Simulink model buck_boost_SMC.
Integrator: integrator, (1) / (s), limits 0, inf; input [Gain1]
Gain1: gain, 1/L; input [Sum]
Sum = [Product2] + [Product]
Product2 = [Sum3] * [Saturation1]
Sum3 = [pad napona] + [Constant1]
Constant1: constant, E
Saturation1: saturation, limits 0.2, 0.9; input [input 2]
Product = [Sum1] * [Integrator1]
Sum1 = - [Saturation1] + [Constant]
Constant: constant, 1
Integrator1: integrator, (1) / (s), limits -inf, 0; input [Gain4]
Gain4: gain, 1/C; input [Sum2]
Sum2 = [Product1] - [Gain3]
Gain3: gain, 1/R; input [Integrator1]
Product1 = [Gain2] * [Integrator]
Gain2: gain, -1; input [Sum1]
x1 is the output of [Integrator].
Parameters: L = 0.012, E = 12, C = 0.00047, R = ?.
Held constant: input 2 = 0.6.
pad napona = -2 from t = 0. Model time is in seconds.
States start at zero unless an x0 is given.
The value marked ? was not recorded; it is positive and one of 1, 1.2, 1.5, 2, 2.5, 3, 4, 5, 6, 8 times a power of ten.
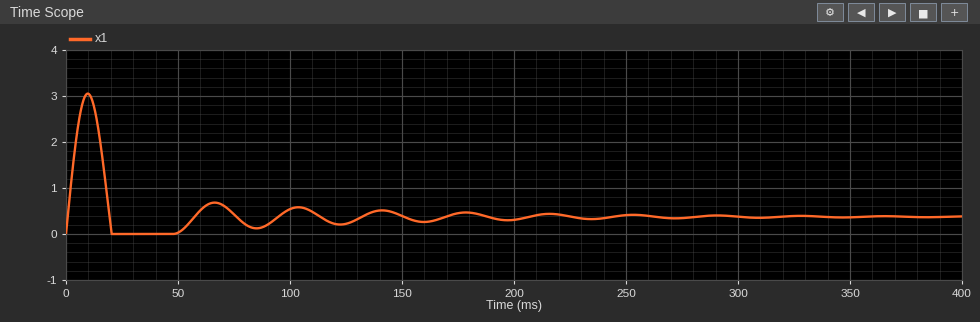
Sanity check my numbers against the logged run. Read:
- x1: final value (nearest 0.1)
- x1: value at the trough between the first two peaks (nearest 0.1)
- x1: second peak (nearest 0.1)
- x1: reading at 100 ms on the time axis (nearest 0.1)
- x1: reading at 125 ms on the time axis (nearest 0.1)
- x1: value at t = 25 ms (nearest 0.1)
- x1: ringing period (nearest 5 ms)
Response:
0.4
0.0
0.7
0.5
0.2
0.0
55 ms
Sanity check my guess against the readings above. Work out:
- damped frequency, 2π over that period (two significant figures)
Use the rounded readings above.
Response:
0.11 rad/ms
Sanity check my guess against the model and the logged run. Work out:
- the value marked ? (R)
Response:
100
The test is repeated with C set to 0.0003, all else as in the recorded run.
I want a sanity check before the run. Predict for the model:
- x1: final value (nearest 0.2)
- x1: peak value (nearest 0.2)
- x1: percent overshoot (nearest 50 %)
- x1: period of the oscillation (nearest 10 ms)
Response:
0.4
2.4
550 %
40 ms
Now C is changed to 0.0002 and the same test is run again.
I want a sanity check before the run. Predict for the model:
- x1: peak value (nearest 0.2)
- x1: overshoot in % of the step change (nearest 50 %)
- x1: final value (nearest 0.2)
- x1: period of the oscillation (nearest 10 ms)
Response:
2.0
450 %
0.4
30 ms
